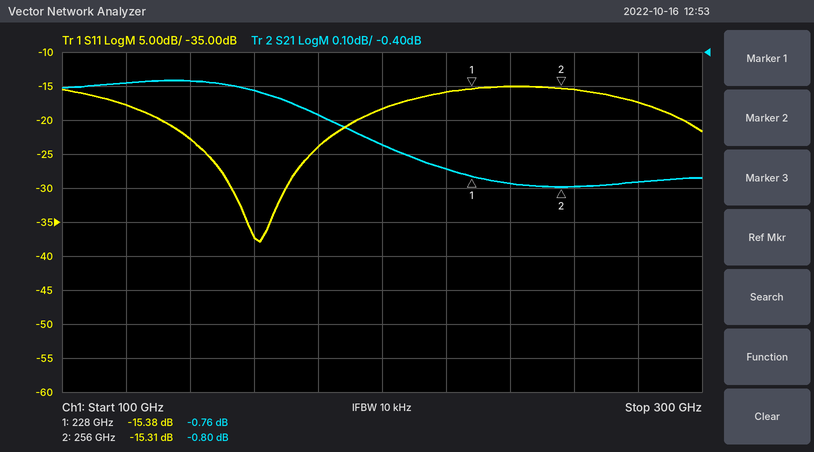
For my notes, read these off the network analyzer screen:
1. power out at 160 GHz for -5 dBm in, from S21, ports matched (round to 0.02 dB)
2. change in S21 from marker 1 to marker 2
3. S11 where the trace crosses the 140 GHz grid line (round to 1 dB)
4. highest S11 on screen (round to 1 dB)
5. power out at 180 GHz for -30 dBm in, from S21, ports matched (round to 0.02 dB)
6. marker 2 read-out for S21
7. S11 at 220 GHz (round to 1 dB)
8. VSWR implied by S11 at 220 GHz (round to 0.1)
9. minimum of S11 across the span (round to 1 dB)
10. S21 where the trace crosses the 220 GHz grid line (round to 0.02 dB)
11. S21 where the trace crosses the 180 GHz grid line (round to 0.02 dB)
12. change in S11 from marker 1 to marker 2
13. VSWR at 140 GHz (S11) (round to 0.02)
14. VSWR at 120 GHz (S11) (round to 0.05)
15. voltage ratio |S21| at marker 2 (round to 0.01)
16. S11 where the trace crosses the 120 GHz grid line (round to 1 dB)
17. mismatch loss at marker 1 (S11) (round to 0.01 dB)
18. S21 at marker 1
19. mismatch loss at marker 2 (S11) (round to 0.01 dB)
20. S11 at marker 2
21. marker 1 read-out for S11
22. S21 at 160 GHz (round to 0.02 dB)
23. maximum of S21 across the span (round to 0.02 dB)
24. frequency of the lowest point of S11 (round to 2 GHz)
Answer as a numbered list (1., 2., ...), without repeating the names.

1. -5.52 dBm
2. -0.04 dB
3. -23 dB
4. -15 dB
5. -30.58 dBm
6. -0.80 dB
7. -16 dB
8. 1.4
9. -38 dB
10. -0.74 dB
11. -0.58 dB
12. 0.07 dB
13. 1.16
14. 1.30
15. 0.91
16. -18 dB
17. 0.13 dB
18. -0.76 dB
19. 0.13 dB
20. -15.31 dB
21. -15.38 dB
22. -0.52 dB
23. -0.48 dB
24. 162 GHz
